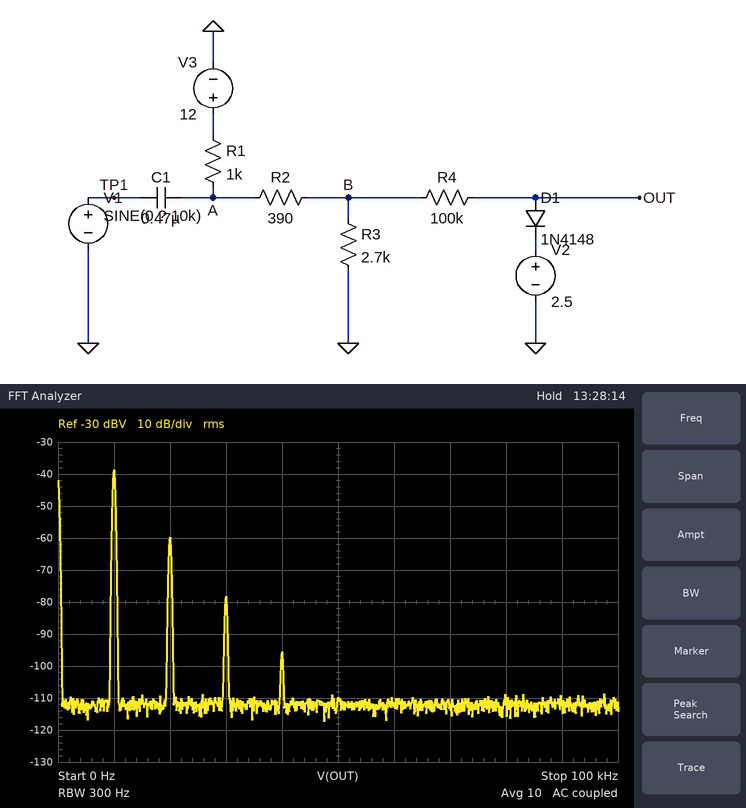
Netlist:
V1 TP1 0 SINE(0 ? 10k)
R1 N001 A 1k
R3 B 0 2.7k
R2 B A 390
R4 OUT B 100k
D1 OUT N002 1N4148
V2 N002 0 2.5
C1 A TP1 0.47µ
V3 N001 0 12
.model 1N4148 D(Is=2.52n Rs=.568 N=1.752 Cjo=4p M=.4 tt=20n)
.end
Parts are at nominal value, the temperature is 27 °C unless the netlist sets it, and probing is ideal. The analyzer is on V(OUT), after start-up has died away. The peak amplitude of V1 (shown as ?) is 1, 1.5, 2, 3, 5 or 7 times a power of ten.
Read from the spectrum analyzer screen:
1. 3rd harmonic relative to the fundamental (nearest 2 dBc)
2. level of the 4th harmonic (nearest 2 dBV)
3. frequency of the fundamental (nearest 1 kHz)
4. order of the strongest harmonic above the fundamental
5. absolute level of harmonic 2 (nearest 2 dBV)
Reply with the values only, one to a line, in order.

-40 dBc
-96 dBV
10 kHz
2
-60 dBV
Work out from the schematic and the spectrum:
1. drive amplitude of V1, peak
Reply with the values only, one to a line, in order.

2 V
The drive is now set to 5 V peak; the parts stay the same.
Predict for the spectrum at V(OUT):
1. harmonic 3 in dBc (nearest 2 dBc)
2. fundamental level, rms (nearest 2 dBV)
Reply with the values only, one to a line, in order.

-20 dBc
-28 dBV
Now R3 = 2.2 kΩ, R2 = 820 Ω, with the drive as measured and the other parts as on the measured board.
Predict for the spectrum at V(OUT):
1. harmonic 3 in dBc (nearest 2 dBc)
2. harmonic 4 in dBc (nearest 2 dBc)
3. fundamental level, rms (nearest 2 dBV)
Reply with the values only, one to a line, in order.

-38 dBc
-54 dBc
-38 dBV
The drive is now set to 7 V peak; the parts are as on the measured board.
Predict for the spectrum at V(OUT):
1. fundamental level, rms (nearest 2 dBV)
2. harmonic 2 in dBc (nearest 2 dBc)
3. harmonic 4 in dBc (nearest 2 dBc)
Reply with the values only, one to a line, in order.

-12 dBV
-2 dBc
-8 dBc
